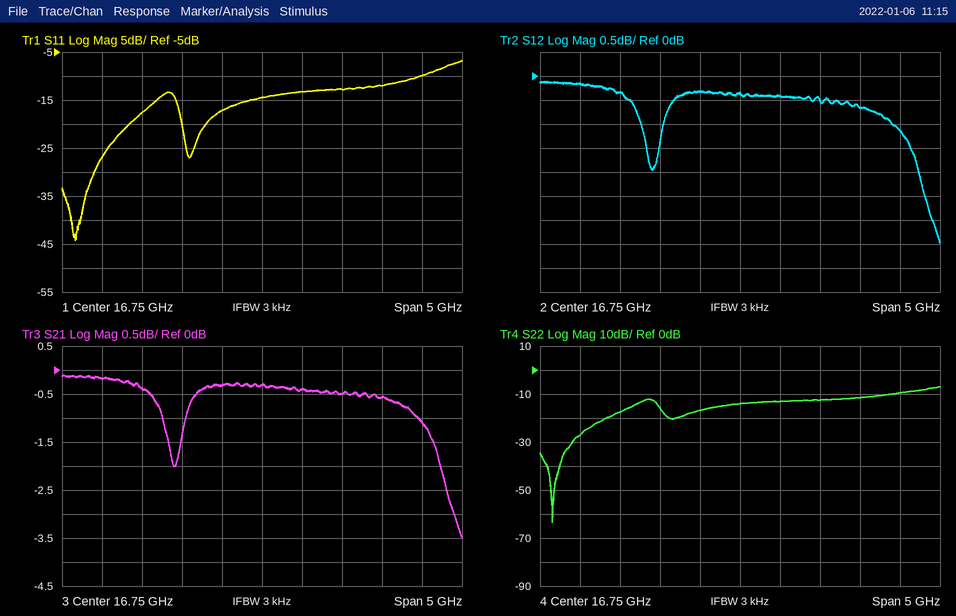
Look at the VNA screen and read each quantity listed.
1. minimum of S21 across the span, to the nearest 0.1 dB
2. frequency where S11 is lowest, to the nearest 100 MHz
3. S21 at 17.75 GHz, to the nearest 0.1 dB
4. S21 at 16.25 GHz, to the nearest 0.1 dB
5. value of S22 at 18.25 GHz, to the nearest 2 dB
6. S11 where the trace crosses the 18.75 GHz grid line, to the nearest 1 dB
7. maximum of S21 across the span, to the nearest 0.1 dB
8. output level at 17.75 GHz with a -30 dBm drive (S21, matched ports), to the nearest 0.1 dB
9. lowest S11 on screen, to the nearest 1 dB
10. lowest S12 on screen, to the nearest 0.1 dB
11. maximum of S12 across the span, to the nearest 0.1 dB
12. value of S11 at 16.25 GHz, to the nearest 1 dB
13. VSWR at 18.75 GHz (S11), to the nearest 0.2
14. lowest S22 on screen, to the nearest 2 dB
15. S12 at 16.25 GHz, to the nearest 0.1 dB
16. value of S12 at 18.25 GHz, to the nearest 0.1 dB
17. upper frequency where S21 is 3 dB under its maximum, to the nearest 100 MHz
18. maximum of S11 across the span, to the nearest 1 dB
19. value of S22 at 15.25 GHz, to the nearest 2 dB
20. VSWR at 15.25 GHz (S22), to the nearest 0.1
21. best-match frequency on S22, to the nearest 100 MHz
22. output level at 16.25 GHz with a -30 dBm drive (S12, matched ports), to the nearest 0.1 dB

-3.5 dB
14.4 GHz
-0.5 dB
-0.3 dB
-12 dB
-10 dB
-0.1 dB
-30.5 dBm
-44 dB
-3.5 dB
-0.1 dB
-17 dB
2.0
-64 dB
-0.3 dB
-0.7 dB
19.2 GHz
-7 dB
-18 dB
1.3
14.4 GHz
-30.3 dBm
